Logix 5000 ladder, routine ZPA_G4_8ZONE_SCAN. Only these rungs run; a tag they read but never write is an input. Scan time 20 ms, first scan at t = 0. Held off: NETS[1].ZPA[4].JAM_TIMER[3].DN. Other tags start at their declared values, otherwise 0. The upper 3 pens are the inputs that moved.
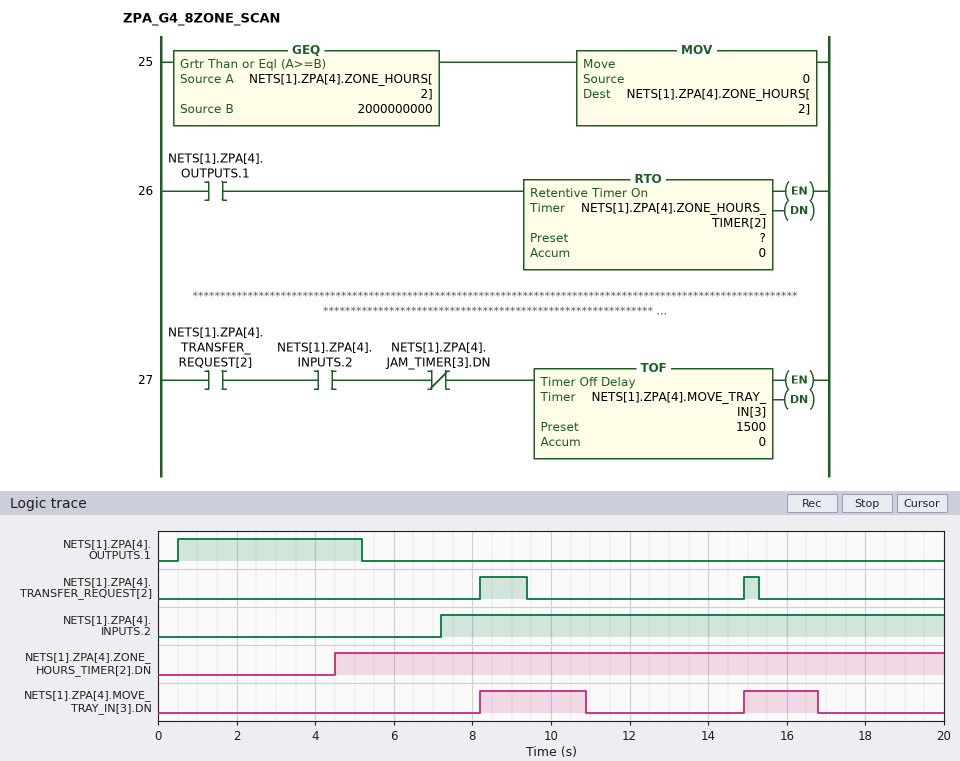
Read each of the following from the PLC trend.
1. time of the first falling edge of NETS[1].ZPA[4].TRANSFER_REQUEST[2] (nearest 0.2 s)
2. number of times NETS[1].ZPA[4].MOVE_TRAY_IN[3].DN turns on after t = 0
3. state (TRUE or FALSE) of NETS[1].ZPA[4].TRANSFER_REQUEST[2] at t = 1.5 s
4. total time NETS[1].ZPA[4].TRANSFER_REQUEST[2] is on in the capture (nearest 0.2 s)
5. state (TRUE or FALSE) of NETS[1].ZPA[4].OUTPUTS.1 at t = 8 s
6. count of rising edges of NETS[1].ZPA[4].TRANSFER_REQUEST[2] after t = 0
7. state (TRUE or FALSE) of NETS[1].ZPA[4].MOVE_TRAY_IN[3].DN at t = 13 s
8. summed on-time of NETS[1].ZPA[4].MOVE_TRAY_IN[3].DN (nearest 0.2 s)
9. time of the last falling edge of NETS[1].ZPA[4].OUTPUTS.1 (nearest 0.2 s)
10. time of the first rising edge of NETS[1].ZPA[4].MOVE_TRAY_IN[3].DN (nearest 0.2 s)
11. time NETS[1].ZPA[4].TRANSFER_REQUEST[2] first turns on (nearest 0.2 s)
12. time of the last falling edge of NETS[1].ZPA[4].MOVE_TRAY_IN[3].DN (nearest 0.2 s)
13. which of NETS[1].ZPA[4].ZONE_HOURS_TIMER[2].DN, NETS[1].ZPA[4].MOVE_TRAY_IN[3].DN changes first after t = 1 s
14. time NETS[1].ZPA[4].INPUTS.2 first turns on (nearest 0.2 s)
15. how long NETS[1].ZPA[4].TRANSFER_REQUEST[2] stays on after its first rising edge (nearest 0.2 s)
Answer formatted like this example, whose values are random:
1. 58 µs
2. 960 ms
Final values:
1. 9.4 s
2. 2
3. FALSE
4. 1.6 s
5. FALSE
6. 2
7. FALSE
8. 4.6 s
9. 5.2 s
10. 8.2 s
11. 8.2 s
12. 16.8 s
13. NETS[1].ZPA[4].ZONE_HOURS_TIMER[2].DN
14. 7.2 s
15. 1.2 s
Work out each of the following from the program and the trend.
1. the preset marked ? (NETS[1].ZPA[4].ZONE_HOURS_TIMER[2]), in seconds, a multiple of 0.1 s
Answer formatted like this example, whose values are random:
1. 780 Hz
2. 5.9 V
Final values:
1. 4.0 s
